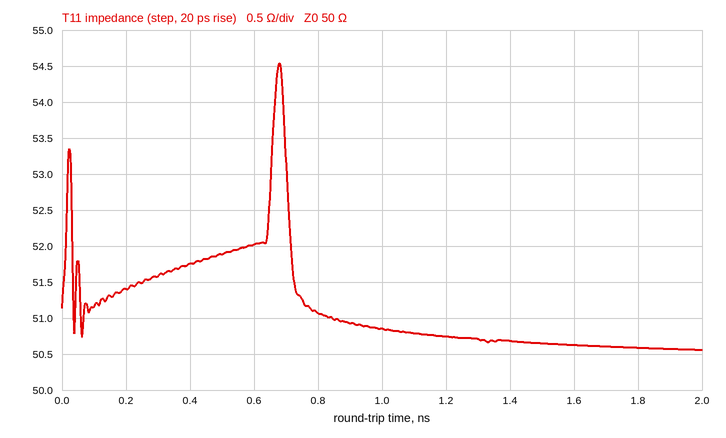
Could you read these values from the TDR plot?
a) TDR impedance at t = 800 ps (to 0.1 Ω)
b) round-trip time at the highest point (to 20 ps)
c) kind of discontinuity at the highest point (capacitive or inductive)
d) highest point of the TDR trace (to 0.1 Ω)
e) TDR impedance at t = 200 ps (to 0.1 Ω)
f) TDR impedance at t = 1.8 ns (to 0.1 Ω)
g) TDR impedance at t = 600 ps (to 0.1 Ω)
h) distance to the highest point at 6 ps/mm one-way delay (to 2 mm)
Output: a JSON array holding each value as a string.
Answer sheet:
["51.1 Ω", "680 ps", "inductive", "54.5 Ω", "51.4 Ω", "50.6 Ω", "52.0 Ω", "56 mm"]
